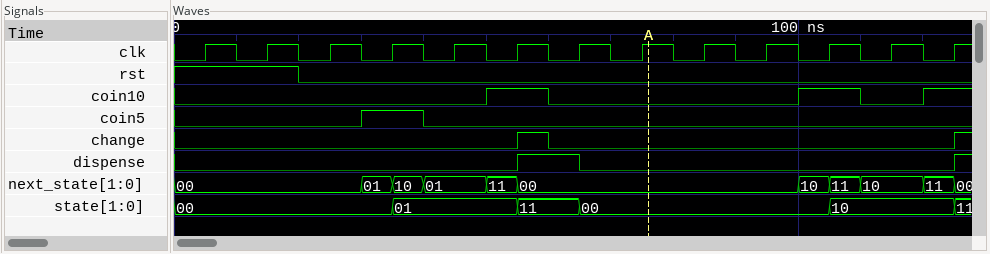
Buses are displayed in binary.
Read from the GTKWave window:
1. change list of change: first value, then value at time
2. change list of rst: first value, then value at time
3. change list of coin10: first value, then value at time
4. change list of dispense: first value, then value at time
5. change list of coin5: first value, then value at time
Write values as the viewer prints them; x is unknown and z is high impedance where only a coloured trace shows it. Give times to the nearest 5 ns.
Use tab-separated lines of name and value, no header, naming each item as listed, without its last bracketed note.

change list of change: first value, then value at time	0, 1 at 55 ns, 0 at 60 ns, 1 at 125 ns
change list of rst: first value, then value at time	1, 0 at 20 ns
change list of coin10: first value, then value at time	0, 1 at 50 ns, 0 at 60 ns, 1 at 100 ns, 0 at 110 ns, 1 at 120 ns
change list of dispense: first value, then value at time	0, 1 at 55 ns, 0 at 65 ns, 1 at 125 ns
change list of coin5: first value, then value at time	0, 1 at 30 ns, 0 at 40 ns
